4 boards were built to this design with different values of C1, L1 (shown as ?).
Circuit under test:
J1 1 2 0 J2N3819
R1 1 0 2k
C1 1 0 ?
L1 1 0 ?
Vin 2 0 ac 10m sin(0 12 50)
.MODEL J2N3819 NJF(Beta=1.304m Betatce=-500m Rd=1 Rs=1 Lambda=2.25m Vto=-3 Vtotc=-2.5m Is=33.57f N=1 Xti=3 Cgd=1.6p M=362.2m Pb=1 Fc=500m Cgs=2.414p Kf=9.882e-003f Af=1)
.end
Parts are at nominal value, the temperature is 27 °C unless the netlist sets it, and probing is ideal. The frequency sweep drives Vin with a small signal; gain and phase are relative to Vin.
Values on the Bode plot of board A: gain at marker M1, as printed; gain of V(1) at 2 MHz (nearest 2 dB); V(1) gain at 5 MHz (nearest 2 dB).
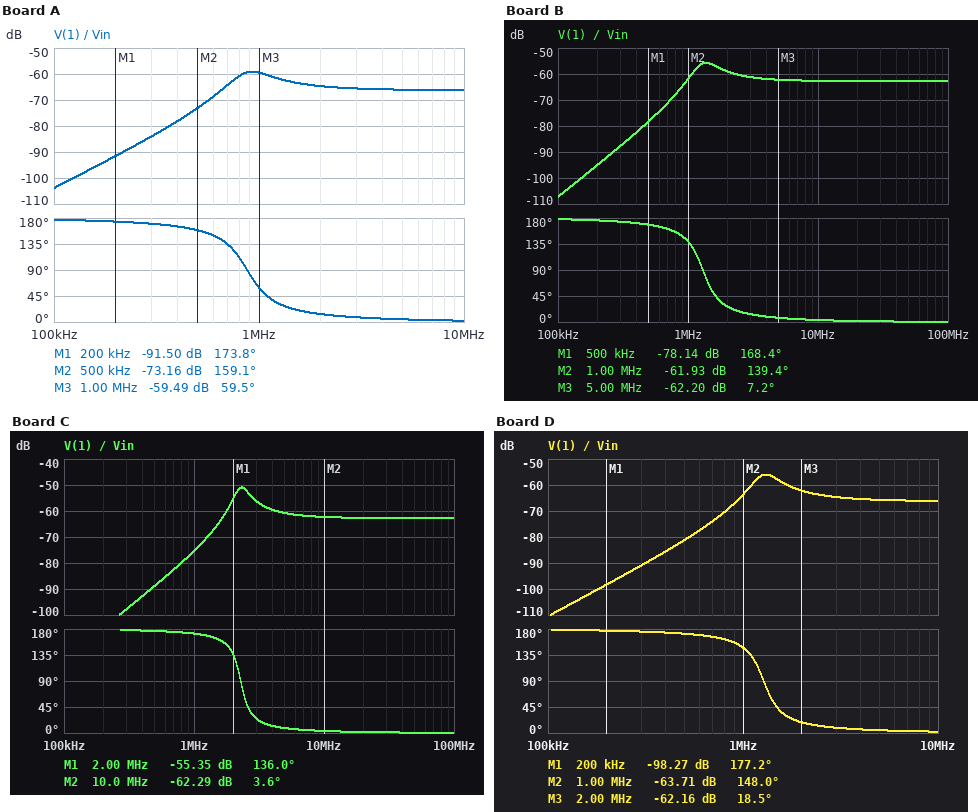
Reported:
-91.50 dB
-64 dB
-66 dB
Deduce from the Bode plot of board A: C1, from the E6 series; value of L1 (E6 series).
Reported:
3.3 nF
10 µH
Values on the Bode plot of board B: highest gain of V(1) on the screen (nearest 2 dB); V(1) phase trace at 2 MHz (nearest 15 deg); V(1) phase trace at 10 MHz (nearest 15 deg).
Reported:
-56 dB
30 deg
0 deg
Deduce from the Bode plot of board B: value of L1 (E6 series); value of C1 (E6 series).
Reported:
6.8 µH
2.2 nF
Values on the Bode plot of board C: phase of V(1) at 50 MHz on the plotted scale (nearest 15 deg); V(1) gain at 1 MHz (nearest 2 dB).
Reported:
0 deg
-76 dB
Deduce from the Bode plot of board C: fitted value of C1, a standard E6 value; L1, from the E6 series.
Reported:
2.2 nF
2.2 µH
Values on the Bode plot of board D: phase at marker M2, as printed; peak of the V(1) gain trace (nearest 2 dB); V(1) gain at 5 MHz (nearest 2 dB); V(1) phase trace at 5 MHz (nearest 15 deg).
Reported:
148.0 deg
-56 dB
-66 dB
0 deg
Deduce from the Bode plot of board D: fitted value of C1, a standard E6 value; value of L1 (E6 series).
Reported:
3.3 nF
4.7 µH
